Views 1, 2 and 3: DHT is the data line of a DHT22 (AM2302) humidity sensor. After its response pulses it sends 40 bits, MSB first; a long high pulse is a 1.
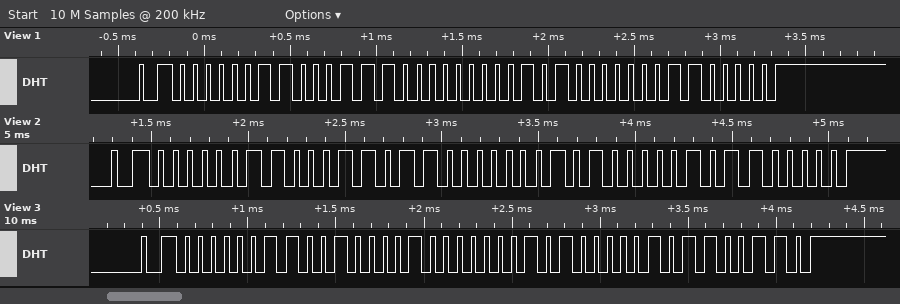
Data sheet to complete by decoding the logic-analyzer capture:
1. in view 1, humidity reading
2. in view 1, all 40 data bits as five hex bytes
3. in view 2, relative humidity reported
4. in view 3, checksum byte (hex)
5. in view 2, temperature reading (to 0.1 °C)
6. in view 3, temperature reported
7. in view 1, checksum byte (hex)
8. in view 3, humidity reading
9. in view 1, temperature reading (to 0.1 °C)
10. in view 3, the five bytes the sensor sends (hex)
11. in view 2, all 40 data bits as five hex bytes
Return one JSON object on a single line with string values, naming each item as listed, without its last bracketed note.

{"in view 1, humidity reading": "79.6 %", "in view 1, all 40 data bits as five hex bytes": "03 1C 01 40 60", "in view 2, relative humidity reported": "79.5 %", "in view 3, checksum byte": "0x66", "in view 2, temperature reading": "32.1 °C", "in view 3, temperature reported": "32.1 °C", "in view 1, checksum byte": "0x60", "in view 3, humidity reading": "80.1 %", "in view 1, temperature reading": "32.0 °C", "in view 3, the five bytes the sensor sends": "03 21 01 41 66", "in view 2, all 40 data bits as five hex bytes": "03 1B 01 41 60"}
